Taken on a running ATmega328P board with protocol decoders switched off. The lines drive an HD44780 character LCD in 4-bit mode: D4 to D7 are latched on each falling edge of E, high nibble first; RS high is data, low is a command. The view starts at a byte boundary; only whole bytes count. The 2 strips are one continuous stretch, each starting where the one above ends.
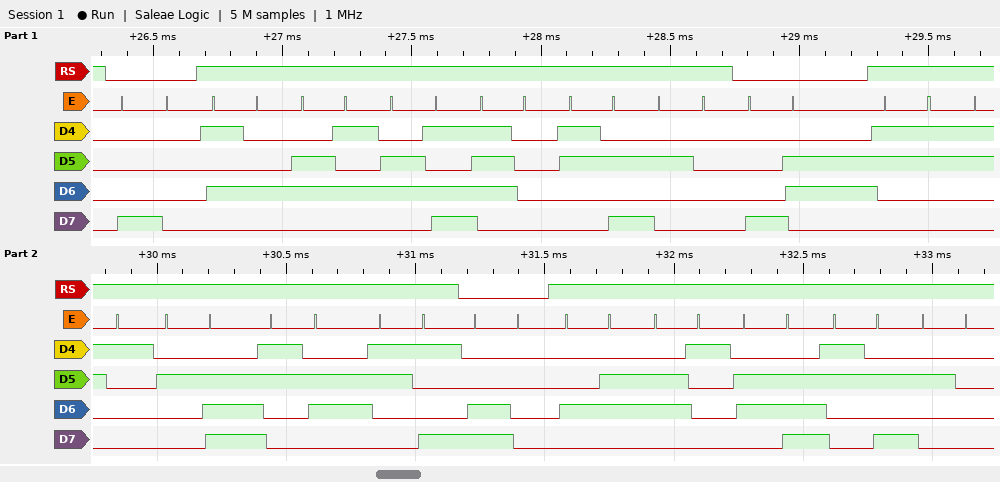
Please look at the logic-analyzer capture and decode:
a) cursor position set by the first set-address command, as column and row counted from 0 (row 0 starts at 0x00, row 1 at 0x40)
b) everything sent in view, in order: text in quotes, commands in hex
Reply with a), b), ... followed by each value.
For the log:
a) column 0, row 0
b) 0x80 "Temp: " 0x86 "31.69" 0xC0 "Fan: "
